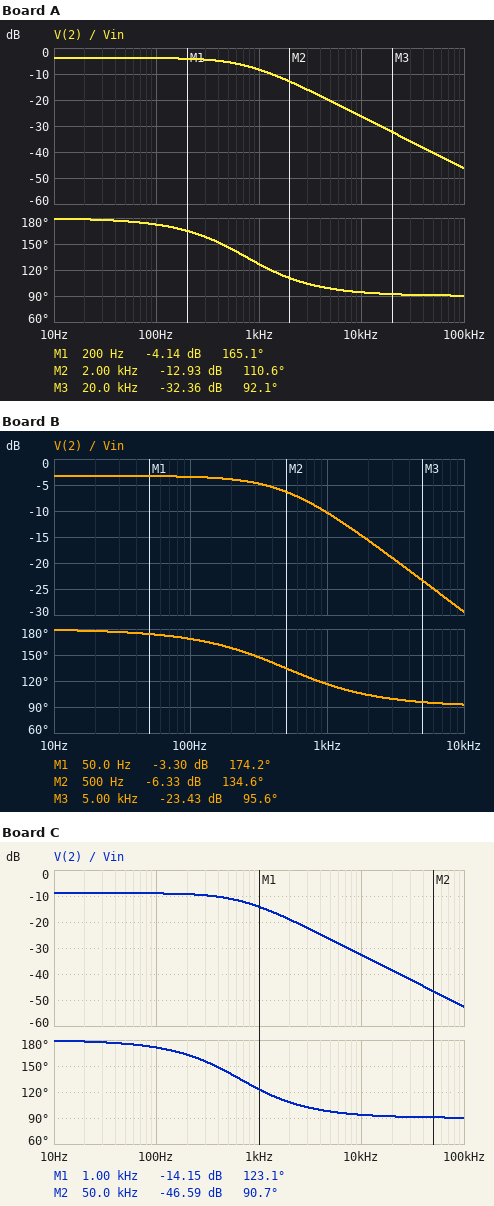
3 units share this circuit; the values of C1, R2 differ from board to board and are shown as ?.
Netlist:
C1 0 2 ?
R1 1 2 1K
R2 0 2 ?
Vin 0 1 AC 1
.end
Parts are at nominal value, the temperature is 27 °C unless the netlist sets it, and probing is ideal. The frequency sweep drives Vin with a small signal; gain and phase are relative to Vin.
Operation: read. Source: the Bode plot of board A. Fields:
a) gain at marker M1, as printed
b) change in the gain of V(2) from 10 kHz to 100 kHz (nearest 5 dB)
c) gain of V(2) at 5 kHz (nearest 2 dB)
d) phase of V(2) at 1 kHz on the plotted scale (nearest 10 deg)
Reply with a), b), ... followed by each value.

a) -4.14 dB
b) -20 dB
c) -20 dB
d) 130 deg
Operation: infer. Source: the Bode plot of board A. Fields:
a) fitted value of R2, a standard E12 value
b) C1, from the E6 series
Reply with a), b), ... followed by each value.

a) 1.8 kΩ
b) 330 nF
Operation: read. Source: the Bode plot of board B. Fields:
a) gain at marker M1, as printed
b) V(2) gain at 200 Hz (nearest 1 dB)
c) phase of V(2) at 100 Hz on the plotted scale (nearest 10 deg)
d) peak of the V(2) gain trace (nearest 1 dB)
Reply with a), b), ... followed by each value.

a) -3.30 dB
b) -4 dB
c) 170 deg
d) -3 dB
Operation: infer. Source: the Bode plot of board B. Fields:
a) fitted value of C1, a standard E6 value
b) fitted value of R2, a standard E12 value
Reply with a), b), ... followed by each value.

a) 470 nF
b) 2.2 kΩ
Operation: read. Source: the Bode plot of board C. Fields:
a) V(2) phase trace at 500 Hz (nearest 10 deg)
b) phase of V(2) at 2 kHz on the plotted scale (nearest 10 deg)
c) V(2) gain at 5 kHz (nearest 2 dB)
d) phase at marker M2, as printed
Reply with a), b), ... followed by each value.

a) 140 deg
b) 110 deg
c) -26 dB
d) 90.7 deg
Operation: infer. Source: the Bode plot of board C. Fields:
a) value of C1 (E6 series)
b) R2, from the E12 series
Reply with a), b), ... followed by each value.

a) 680 nF
b) 560 Ω
